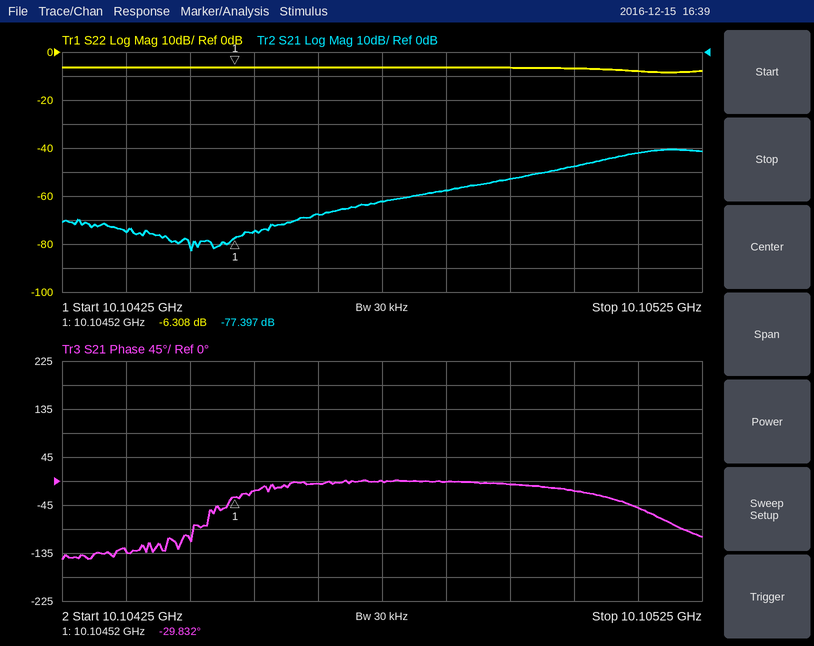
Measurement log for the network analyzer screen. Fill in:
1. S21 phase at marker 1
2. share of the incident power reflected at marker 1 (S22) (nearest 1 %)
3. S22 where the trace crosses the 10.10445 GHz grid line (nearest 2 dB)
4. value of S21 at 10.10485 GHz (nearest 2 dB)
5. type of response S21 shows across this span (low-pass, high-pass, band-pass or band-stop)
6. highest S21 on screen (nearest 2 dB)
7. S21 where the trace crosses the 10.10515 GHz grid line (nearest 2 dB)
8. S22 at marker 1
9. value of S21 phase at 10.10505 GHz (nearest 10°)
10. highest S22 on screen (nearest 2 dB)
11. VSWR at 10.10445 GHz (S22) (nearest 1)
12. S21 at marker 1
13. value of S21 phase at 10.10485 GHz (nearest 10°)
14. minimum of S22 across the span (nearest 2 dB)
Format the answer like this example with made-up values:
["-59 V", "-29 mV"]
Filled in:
["-29.832°", "23 %", "-6 dB", "-58 dB", "high-pass", "-40 dB", "-42 dB", "-6.308 dB", "-20°", "-6 dB", "3", "-77.397 dB", "0°", "-8 dB"]
